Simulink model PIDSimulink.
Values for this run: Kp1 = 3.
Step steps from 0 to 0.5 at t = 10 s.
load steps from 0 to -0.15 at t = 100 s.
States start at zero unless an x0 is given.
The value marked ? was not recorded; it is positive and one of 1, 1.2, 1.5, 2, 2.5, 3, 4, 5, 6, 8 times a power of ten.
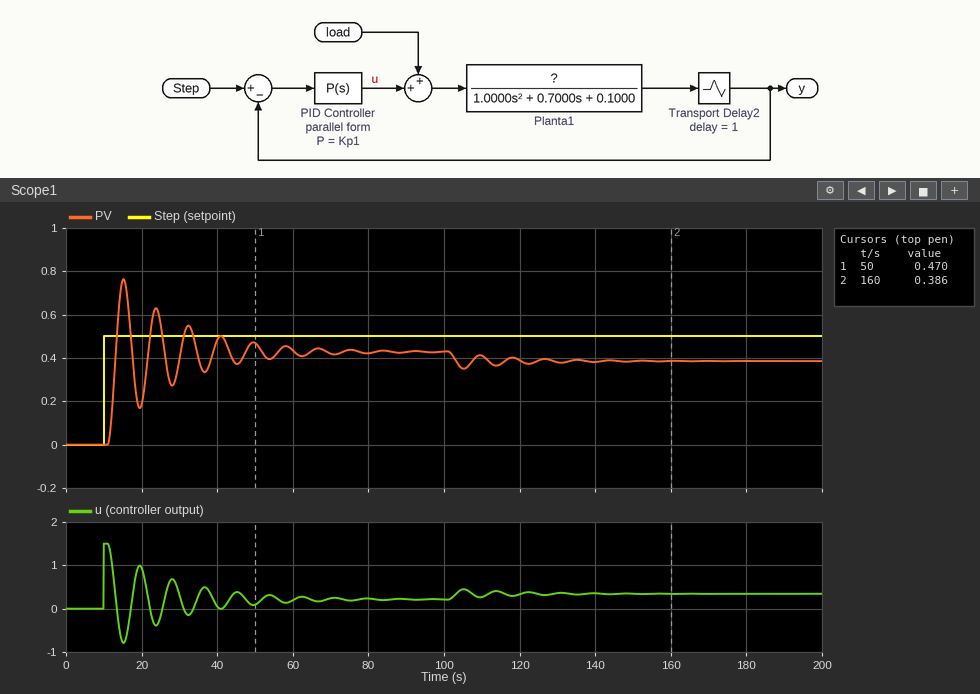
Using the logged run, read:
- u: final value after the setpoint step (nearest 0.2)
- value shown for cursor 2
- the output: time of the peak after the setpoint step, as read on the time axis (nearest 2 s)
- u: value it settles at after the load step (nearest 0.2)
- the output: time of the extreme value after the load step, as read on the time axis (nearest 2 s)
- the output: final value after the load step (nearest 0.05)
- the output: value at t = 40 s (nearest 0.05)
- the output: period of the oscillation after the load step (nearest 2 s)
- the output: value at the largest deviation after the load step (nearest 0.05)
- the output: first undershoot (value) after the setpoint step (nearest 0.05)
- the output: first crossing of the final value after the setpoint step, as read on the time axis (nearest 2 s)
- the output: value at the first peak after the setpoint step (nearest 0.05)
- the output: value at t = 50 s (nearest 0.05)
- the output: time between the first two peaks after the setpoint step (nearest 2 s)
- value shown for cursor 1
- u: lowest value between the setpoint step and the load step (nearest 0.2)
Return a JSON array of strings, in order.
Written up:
["0.2", "0.386", "16 s", "0.4", "106 s", "0.40", "0.50", "8 s", "0.35", "0.15", "14 s", "0.75", "0.45", "8 s", "0.470", "-0.8"]
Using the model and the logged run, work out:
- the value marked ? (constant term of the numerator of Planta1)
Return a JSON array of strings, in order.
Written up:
["0.2"]
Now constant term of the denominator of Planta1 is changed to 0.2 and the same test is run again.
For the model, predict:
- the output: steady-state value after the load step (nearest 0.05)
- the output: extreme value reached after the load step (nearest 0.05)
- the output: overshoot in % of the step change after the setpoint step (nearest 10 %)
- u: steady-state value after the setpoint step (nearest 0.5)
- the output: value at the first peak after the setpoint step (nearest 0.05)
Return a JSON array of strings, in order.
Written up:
["0.35", "0.30", "80 %", "0.5", "0.65"]
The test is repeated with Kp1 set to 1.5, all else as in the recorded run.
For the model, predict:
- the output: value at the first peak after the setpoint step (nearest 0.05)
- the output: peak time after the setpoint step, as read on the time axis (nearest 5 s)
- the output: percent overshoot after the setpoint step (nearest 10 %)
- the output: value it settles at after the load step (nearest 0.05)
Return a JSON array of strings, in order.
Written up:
["0.50", "15 s", "40 %", "0.30"]
